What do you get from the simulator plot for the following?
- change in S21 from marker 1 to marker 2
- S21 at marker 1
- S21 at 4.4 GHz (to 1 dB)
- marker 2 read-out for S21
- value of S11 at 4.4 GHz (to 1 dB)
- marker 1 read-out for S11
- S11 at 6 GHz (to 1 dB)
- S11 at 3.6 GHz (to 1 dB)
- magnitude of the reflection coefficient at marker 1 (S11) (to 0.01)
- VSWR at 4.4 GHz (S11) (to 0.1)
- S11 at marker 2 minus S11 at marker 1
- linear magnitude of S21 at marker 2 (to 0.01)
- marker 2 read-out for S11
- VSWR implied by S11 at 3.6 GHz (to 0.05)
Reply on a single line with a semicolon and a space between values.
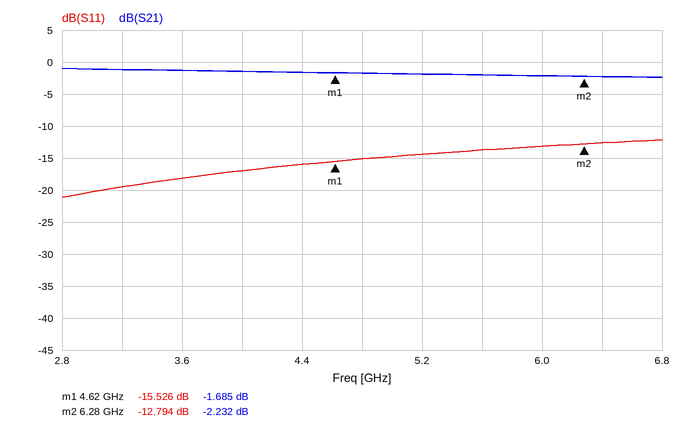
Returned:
-0.547 dB; -1.685 dB; -2 dB; -2.232 dB; -16 dB; -15.526 dB; -13 dB; -18 dB; 0.17; 1.4; 2.732 dB; 0.77; -12.794 dB; 1.30
